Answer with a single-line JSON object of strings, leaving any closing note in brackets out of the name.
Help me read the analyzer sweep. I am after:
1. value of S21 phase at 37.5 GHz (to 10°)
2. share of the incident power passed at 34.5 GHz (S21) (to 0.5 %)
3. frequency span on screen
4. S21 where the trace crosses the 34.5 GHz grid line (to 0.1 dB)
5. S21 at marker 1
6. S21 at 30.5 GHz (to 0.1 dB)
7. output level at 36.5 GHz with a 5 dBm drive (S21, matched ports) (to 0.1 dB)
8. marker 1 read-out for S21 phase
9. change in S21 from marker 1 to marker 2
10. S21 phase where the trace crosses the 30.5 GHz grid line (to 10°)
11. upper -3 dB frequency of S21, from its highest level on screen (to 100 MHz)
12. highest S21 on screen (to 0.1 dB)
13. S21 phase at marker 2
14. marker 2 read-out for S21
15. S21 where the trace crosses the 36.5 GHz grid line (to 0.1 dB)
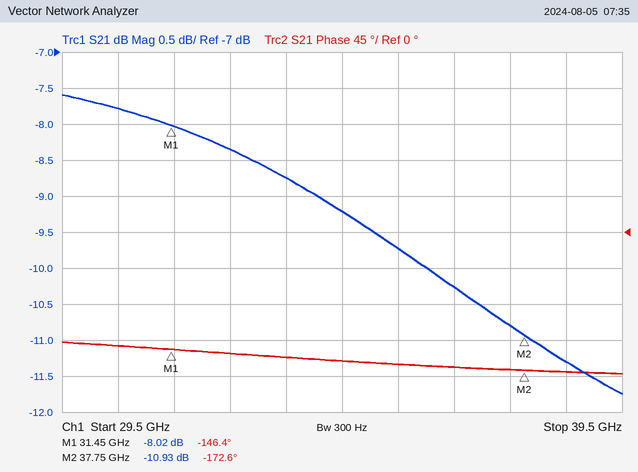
{"value of S21 phase at 37.5 GHz": "-170°", "share of the incident power passed at 34.5 GHz (S21)": "12.0 %", "frequency span on screen": "10 GHz", "S21 where the trace crosses the 34.5 GHz grid line": "-9.2 dB", "S21 at marker 1": "-8.02 dB", "S21 at 30.5 GHz": "-7.8 dB", "output level at 36.5 GHz with a 5 dBm drive (S21, matched ports)": "-5.3 dBm", "marker 1 read-out for S21 phase": "-146.4°", "change in S21 from marker 1 to marker 2": "-2.91 dB", "S21 phase where the trace crosses the 30.5 GHz grid line": "-140°", "upper -3 dB frequency of S21, from its highest level on screen": "37.1 GHz", "highest S21 on screen": "-7.6 dB", "S21 phase at marker 2": "-172.6°", "marker 2 read-out for S21": "-10.93 dB", "S21 where the trace crosses the 36.5 GHz grid line": "-10.3 dB"}
